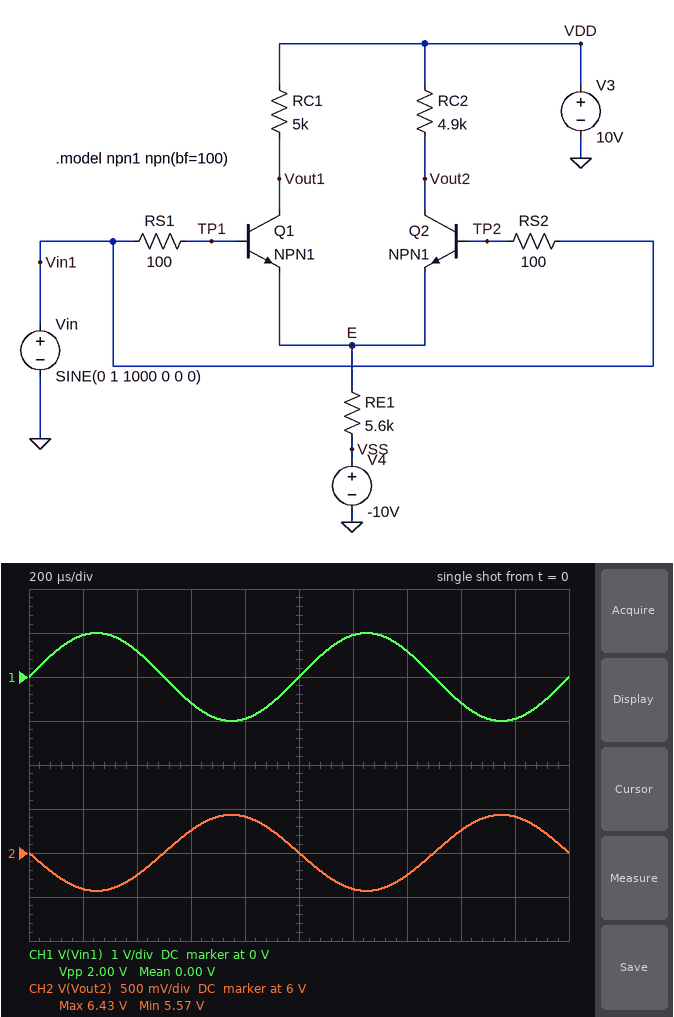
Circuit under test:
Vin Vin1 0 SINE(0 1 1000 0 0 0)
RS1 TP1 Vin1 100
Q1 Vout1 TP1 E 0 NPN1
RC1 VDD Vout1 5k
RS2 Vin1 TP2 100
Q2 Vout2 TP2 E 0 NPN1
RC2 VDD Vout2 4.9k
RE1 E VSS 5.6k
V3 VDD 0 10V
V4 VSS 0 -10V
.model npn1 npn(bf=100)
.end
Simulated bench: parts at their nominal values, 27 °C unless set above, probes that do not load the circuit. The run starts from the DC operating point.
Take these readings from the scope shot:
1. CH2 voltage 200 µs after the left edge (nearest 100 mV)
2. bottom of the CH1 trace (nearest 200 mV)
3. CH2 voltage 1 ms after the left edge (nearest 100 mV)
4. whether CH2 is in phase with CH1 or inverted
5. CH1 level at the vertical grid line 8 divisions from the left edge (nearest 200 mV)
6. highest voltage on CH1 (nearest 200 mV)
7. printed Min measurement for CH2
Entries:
5.6 V
-1.0 V
6.0 V
inverted
-600 mV
1.0 V
5.57 V
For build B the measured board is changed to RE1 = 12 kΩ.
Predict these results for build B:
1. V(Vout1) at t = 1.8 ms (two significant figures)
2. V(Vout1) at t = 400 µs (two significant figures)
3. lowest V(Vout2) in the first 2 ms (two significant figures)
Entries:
8.3 V
8.0 V
7.9 V
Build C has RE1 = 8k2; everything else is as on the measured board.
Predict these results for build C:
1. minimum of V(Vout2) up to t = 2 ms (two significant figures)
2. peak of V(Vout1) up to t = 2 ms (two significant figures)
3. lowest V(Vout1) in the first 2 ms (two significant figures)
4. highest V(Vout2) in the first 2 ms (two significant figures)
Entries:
7.0 V
7.5 V
6.9 V
7.6 V
